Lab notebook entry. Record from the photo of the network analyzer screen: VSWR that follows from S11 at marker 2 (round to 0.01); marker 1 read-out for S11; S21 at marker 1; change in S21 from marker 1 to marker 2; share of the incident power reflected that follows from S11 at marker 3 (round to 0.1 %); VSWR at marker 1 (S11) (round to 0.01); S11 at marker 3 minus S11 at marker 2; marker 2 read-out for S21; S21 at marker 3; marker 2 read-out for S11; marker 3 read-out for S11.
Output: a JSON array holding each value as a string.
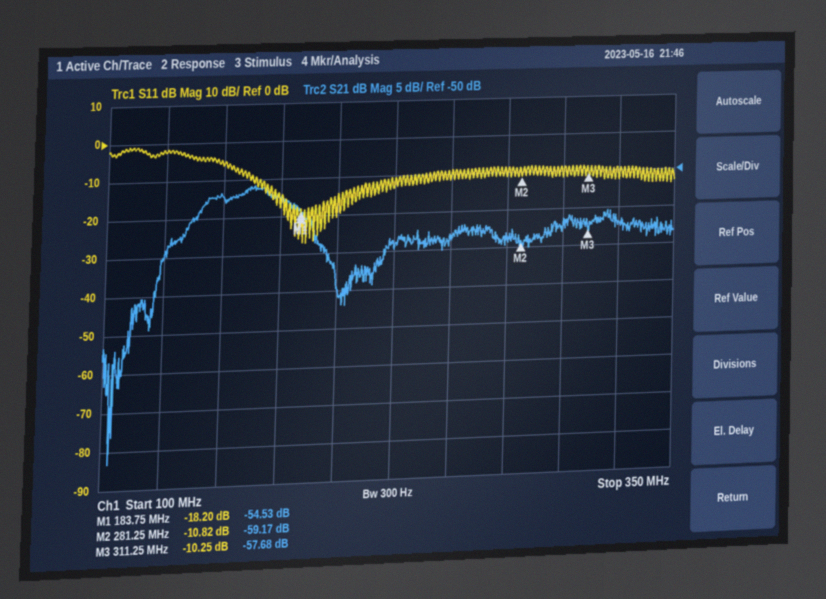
["1.81", "-18.20 dB", "-54.53 dB", "-4.64 dB", "9.4 %", "1.28", "0.57 dB", "-59.17 dB", "-57.68 dB", "-10.82 dB", "-10.25 dB"]
